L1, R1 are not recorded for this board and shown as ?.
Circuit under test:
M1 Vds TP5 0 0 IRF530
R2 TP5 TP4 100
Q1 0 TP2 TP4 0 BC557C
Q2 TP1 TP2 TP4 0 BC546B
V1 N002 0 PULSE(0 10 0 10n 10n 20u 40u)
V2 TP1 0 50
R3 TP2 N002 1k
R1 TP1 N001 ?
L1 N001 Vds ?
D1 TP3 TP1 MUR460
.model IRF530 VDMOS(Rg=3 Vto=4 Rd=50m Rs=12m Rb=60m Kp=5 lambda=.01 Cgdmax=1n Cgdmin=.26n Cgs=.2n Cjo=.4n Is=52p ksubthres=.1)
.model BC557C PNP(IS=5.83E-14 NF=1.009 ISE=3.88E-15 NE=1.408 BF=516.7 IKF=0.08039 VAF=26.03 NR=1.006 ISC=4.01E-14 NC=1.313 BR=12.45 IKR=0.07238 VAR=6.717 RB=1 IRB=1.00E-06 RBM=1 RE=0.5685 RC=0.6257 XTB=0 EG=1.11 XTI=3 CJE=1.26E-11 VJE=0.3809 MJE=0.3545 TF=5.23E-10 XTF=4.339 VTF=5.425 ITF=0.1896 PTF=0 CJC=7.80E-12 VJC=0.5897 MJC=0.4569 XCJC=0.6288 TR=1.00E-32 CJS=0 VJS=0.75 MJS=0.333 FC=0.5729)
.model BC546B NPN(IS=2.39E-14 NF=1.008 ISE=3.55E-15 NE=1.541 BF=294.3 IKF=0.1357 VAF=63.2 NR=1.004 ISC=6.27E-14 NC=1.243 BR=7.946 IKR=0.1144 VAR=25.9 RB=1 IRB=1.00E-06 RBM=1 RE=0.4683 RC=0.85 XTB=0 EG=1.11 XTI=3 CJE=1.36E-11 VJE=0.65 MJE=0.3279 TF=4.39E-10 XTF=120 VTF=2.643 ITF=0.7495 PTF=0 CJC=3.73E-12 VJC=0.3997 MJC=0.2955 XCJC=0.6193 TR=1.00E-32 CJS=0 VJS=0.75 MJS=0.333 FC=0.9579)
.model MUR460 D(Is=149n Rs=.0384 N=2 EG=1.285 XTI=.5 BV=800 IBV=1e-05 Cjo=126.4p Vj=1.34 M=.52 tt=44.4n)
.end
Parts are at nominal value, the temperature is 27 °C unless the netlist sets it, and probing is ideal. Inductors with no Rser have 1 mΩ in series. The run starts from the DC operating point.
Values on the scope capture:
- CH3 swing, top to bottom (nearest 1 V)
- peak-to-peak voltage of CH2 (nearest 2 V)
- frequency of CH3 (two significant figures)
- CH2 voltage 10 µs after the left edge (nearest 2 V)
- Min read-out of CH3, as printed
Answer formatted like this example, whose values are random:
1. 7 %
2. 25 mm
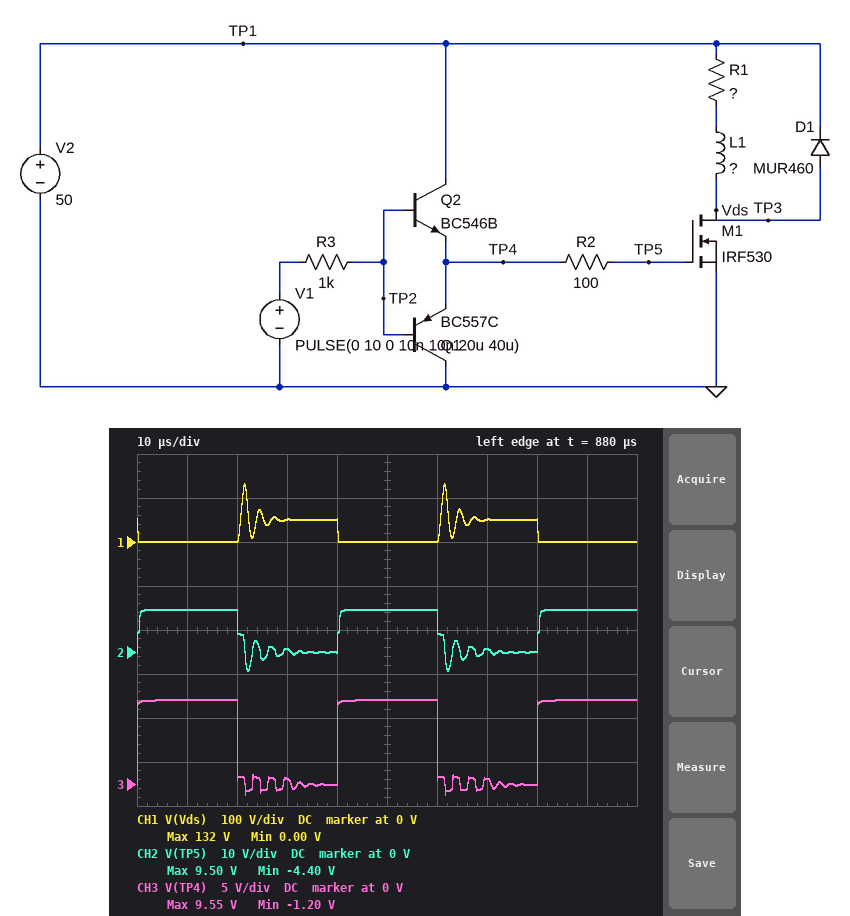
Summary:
1. 11 V
2. 14 V
3. 25 kHz
4. 10 V
5. -1.20 V
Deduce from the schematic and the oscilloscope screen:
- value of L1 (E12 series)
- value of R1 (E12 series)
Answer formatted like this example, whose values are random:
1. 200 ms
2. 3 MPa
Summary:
1. 680 µH
2. 470 Ω
